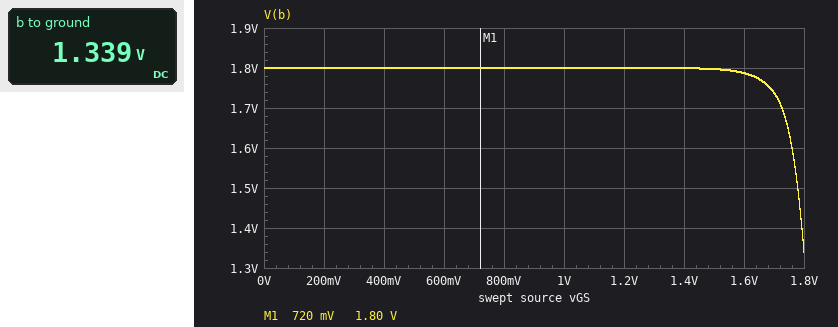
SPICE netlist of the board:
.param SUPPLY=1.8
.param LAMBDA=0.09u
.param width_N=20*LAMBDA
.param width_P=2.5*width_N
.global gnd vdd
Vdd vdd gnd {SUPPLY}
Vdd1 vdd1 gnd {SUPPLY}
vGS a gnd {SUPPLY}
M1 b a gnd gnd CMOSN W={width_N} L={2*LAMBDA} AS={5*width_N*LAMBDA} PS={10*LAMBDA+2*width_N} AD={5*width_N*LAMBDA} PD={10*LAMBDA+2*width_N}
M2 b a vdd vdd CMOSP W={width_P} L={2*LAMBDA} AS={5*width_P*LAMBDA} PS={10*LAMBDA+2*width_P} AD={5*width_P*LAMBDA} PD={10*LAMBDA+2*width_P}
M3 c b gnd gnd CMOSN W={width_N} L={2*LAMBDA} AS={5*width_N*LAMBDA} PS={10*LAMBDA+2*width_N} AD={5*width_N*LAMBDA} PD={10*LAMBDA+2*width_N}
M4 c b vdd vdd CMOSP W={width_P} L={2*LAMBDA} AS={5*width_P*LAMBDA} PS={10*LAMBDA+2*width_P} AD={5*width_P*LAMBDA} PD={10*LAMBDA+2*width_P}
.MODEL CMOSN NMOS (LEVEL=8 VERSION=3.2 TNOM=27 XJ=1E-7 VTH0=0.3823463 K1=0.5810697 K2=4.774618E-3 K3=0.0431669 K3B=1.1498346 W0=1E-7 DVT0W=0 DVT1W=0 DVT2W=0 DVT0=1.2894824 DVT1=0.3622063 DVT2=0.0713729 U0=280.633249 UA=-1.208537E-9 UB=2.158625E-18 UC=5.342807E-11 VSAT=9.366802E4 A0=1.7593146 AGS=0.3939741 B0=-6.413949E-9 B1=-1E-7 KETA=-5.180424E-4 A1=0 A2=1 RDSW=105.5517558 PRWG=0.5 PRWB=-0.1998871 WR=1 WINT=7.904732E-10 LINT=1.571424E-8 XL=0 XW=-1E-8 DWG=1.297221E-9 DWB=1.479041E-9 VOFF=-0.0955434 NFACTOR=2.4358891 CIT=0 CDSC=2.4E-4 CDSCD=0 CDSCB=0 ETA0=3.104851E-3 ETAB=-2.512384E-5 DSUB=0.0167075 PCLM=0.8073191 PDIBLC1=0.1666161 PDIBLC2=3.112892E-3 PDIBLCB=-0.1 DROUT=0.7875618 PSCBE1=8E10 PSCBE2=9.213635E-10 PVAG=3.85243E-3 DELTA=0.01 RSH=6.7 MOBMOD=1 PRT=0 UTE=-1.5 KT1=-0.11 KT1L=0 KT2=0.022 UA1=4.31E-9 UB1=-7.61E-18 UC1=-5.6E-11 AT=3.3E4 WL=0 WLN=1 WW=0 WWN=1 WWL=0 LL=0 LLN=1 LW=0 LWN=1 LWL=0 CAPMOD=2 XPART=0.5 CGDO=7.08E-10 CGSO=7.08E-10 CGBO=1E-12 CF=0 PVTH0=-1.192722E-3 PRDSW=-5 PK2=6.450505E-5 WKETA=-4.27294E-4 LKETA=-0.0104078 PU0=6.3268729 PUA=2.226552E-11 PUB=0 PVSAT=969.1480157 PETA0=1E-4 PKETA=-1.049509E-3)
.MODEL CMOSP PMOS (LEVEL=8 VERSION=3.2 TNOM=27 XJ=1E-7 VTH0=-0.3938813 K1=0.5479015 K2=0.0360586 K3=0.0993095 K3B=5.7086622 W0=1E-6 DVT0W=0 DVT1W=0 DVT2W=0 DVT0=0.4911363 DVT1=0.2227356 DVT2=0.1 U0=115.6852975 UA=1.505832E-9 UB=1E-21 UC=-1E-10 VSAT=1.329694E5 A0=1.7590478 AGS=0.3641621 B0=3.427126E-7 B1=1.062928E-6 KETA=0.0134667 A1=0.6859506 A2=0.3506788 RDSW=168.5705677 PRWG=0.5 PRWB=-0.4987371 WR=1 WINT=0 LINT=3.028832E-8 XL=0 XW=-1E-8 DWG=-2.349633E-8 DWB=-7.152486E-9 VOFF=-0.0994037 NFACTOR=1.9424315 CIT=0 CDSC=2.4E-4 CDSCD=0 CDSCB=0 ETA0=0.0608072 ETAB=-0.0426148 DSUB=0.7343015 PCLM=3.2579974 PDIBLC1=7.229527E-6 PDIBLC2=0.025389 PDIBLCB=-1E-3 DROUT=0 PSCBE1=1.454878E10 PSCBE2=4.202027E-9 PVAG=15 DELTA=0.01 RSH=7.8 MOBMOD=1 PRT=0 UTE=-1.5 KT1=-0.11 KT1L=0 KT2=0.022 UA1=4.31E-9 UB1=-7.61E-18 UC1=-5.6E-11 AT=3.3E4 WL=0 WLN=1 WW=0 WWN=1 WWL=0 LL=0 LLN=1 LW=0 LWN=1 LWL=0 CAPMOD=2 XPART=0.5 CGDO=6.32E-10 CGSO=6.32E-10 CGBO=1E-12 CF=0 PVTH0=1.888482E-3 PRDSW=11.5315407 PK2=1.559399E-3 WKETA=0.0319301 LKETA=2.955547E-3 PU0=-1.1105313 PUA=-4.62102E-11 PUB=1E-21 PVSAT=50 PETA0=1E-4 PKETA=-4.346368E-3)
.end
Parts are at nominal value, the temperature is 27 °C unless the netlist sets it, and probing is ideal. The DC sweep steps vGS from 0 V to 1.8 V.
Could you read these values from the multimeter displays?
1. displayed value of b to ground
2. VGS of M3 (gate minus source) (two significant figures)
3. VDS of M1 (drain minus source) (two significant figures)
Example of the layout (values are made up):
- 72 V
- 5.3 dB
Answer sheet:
- 1.339 V
- 1.3 V
- 1.3 V
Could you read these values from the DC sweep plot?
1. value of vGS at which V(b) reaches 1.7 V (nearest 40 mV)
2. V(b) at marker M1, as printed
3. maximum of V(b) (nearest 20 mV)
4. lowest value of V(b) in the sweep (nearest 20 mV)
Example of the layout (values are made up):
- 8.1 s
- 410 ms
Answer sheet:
- 1.72 V
- 1.80 V
- 1.80 V
- 1.34 V
